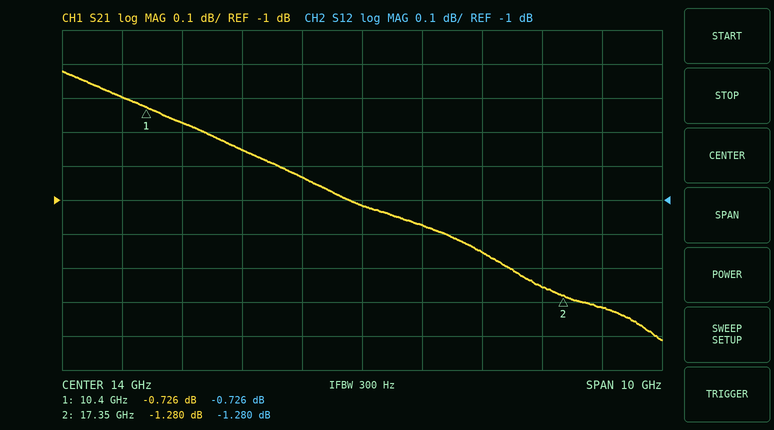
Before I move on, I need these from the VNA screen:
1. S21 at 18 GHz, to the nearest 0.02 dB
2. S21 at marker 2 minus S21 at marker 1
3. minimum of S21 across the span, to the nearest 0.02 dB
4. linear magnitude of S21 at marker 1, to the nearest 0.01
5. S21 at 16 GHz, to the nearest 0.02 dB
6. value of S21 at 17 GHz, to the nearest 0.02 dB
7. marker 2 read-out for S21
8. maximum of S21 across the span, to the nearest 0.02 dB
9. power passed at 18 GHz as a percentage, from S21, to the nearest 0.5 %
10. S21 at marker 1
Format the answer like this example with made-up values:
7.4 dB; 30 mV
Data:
-1.32 dB; -0.554 dB; -1.42 dB; 0.92; -1.16 dB; -1.26 dB; -1.280 dB; -0.62 dB; 74.0 %; -0.726 dB
